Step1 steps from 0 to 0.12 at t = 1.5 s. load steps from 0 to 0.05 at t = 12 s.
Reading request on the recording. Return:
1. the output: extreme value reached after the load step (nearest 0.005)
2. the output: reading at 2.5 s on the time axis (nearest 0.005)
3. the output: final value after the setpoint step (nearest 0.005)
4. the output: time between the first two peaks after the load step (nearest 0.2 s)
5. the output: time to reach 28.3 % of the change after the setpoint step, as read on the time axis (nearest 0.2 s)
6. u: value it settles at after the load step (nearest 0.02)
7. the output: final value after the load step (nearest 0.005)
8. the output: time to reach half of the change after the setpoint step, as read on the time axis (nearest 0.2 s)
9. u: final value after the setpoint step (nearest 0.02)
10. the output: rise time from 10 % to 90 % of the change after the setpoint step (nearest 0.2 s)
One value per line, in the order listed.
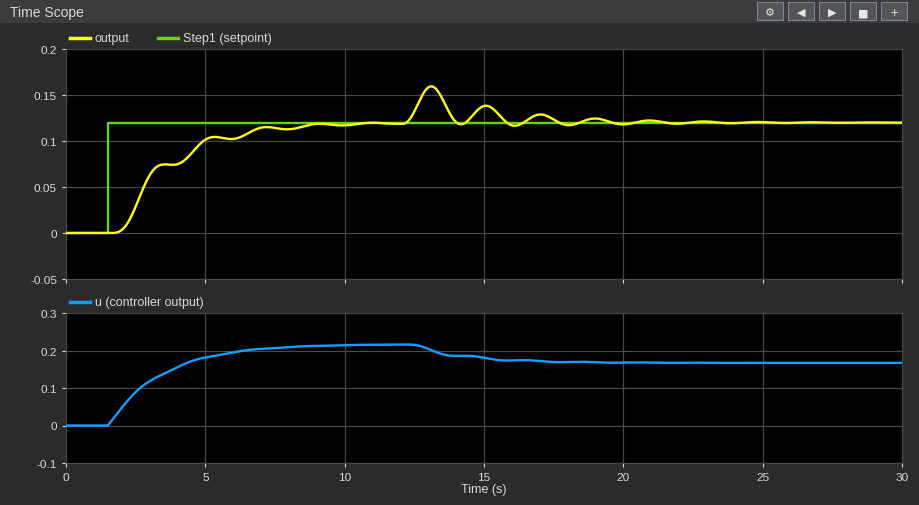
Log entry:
0.160
0.030
0.120
2.0 s
2.6 s
0.16
0.120
3.0 s
0.22
4.2 s
